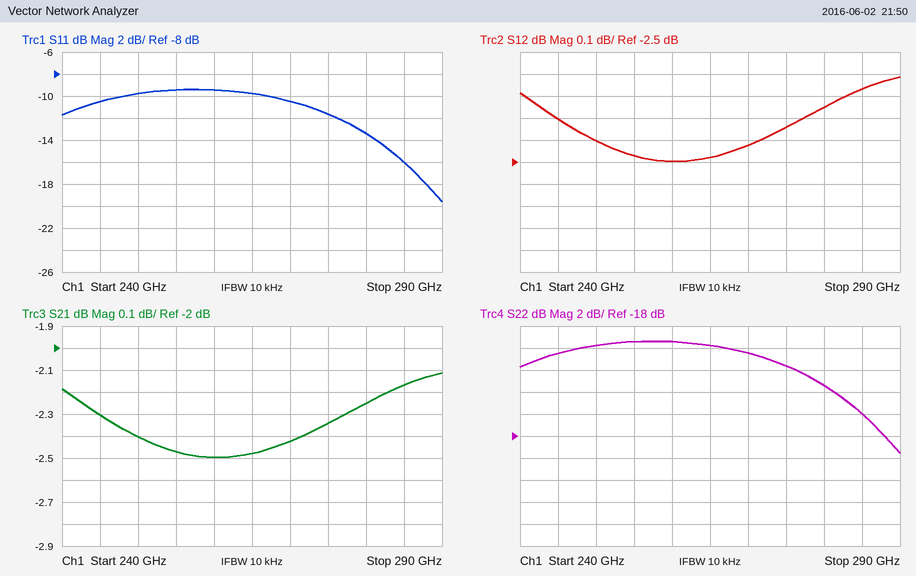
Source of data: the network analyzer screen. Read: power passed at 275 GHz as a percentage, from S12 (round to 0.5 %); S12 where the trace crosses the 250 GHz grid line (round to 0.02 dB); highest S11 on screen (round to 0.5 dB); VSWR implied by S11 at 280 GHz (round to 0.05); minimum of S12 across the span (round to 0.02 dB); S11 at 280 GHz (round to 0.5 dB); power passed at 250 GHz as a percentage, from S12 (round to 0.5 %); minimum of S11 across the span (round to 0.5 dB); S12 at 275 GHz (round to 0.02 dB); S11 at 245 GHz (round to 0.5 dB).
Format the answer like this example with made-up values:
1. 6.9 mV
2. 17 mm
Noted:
1. 58.5 %
2. -2.40 dB
3. -9.5 dB
4. 1.55
5. -2.50 dB
6. -13.5 dB
7. 57.5 %
8. -19.5 dB
9. -2.34 dB
10. -10.5 dB
